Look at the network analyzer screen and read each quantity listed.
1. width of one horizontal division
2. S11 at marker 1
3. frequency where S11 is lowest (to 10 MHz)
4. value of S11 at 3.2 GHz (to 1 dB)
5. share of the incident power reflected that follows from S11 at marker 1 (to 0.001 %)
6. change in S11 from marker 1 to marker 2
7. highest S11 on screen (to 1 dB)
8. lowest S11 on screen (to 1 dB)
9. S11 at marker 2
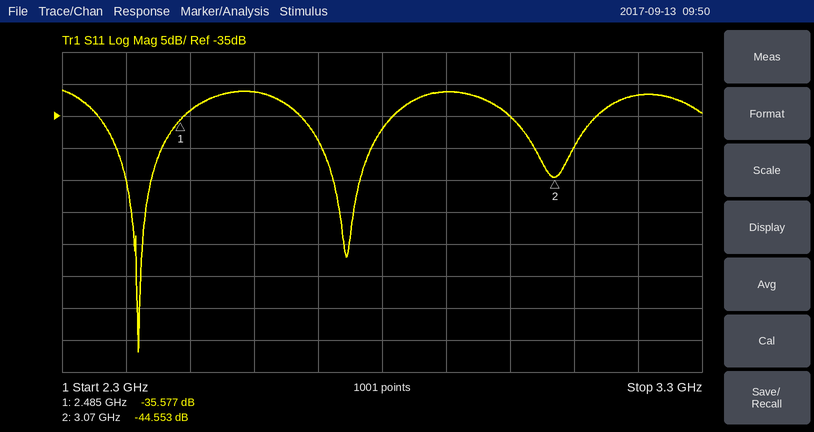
100 MHz
-35.577 dB
2.42 GHz
-32 dB
0.028 %
-8.976 dB
-31 dB
-72 dB
-44.553 dB
